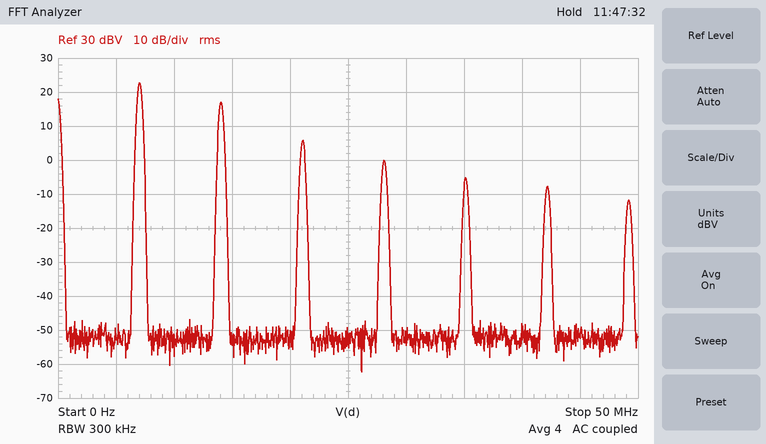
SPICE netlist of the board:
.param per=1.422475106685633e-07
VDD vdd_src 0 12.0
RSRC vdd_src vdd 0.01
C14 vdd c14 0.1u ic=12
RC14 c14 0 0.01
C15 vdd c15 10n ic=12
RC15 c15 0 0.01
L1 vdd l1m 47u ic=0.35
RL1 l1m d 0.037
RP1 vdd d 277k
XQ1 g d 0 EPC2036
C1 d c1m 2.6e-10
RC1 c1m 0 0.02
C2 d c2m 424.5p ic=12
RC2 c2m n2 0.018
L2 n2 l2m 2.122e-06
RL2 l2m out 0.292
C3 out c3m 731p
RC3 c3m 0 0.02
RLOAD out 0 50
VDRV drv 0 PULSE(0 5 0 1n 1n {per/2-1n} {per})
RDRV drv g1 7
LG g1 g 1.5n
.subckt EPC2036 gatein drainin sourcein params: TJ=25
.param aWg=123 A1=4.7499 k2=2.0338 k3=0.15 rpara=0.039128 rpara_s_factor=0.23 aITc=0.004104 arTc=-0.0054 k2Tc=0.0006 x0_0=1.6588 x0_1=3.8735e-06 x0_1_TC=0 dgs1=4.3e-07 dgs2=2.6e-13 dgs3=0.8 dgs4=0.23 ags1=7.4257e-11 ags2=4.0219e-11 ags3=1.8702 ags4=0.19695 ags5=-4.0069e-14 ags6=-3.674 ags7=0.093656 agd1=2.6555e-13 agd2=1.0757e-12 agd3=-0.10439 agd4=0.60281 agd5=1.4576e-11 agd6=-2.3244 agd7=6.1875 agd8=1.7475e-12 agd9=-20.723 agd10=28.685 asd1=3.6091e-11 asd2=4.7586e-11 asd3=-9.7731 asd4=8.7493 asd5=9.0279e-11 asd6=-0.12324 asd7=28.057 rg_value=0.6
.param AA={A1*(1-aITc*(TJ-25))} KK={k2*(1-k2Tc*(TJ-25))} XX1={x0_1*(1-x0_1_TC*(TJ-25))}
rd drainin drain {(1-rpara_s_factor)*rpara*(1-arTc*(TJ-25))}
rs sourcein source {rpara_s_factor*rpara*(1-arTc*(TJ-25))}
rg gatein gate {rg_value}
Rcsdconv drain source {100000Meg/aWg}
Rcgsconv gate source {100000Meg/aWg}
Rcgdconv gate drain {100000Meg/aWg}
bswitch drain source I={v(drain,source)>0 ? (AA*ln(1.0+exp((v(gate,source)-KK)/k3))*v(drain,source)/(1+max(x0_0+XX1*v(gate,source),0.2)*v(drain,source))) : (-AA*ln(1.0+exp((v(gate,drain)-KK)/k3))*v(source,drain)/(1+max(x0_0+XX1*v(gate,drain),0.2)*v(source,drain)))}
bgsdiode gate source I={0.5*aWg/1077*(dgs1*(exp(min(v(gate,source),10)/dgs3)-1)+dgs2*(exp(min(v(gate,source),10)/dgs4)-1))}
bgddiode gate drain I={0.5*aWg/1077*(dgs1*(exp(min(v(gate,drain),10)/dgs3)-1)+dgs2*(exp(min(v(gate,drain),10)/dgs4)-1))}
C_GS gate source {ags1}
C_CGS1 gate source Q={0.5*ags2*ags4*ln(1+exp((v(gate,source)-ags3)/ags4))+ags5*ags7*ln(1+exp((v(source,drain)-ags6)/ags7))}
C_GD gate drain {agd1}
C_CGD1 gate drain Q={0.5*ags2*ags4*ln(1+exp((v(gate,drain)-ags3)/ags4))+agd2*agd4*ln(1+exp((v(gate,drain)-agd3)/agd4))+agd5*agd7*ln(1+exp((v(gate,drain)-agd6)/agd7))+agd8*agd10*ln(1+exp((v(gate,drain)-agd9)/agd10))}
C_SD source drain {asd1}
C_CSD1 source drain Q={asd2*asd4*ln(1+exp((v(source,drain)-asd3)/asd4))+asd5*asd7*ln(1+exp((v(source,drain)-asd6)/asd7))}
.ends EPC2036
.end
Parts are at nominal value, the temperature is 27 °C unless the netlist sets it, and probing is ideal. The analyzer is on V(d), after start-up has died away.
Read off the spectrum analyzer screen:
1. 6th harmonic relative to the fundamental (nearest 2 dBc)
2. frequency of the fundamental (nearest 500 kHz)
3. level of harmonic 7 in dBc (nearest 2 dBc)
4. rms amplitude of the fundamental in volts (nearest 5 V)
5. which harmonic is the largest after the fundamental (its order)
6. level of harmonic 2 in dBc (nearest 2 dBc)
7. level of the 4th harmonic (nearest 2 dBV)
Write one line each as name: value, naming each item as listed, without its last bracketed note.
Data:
6th harmonic relative to the fundamental: -30 dBc
frequency of the fundamental: 7.0 MHz
level of harmonic 7 in dBc: -34 dBc
rms amplitude of the fundamental in volts: 15 V
which harmonic is the largest after the fundamental: 2
level of harmonic 2 in dBc: -6 dBc
level of the 4th harmonic: 0 dBV
